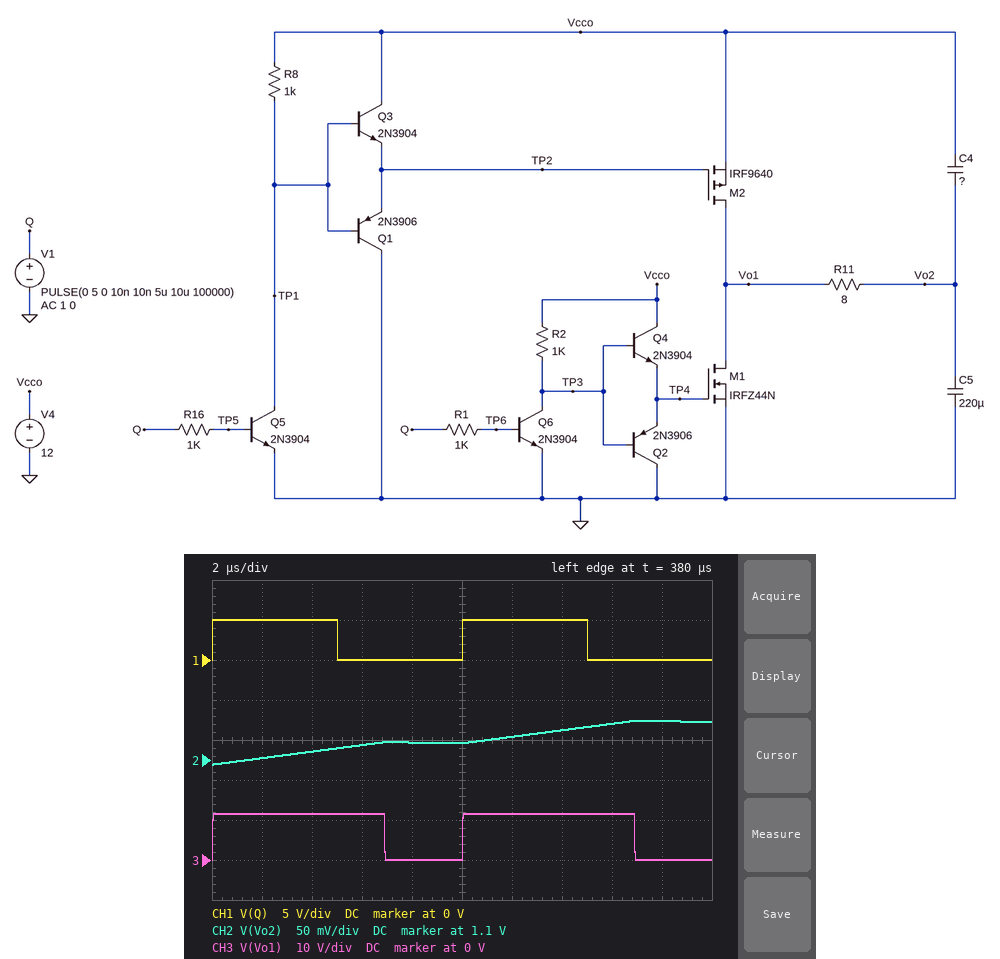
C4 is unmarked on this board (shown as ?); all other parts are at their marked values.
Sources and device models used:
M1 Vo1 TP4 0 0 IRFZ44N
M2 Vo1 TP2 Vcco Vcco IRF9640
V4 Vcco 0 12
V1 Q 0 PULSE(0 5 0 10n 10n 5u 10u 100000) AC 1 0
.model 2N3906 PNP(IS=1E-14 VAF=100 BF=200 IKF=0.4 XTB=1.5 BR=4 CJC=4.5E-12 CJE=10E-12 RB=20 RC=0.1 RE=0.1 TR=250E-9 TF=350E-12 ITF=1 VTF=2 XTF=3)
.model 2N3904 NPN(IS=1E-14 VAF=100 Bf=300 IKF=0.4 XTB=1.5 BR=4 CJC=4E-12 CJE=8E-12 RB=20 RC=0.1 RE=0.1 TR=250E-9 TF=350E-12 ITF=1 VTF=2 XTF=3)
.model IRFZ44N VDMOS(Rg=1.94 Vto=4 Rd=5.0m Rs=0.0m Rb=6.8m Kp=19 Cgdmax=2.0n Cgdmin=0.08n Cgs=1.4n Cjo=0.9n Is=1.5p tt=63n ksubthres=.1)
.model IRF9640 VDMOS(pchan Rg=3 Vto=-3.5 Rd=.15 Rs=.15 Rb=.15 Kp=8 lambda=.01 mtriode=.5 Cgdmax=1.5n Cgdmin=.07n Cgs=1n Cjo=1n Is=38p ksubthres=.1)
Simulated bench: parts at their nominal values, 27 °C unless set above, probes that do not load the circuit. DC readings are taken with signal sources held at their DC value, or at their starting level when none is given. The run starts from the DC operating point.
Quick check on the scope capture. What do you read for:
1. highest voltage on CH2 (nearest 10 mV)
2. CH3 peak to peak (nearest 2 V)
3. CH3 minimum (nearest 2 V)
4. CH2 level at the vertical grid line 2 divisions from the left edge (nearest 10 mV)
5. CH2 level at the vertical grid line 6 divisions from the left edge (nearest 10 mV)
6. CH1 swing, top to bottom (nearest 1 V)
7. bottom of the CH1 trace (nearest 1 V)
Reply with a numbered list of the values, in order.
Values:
1. 1.15 V
2. 12 V
3. 0 V
4. 1.11 V
5. 1.13 V
6. 5 V
7. 0 V
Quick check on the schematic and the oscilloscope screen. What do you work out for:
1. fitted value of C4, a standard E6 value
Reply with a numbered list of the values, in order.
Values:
1. 100 µF
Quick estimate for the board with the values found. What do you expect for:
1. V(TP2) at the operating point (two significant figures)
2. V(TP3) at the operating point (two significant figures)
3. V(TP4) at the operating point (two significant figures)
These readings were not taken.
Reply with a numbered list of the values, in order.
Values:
1. 12 V
2. 12 V
3. 12 V
